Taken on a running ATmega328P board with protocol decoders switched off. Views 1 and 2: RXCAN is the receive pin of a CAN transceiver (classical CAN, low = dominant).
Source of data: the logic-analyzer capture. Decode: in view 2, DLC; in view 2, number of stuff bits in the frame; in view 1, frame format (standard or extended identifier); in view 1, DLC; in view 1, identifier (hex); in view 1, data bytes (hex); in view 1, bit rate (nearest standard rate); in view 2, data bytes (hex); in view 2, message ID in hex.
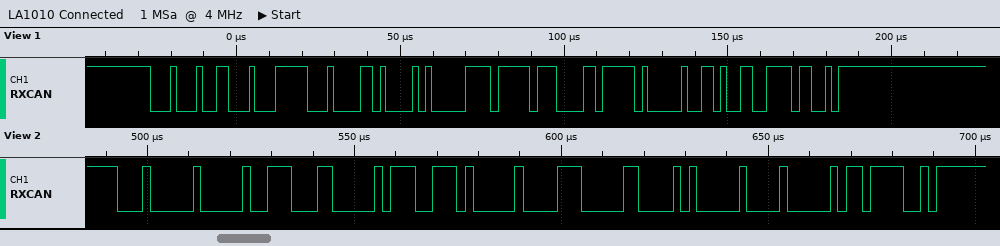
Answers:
7
7
standard
8
0x113
F9 0D 0A 0E FF 0D F8 0D
500 kbit/s
18 1C E8 03 82 14 01
0x100
